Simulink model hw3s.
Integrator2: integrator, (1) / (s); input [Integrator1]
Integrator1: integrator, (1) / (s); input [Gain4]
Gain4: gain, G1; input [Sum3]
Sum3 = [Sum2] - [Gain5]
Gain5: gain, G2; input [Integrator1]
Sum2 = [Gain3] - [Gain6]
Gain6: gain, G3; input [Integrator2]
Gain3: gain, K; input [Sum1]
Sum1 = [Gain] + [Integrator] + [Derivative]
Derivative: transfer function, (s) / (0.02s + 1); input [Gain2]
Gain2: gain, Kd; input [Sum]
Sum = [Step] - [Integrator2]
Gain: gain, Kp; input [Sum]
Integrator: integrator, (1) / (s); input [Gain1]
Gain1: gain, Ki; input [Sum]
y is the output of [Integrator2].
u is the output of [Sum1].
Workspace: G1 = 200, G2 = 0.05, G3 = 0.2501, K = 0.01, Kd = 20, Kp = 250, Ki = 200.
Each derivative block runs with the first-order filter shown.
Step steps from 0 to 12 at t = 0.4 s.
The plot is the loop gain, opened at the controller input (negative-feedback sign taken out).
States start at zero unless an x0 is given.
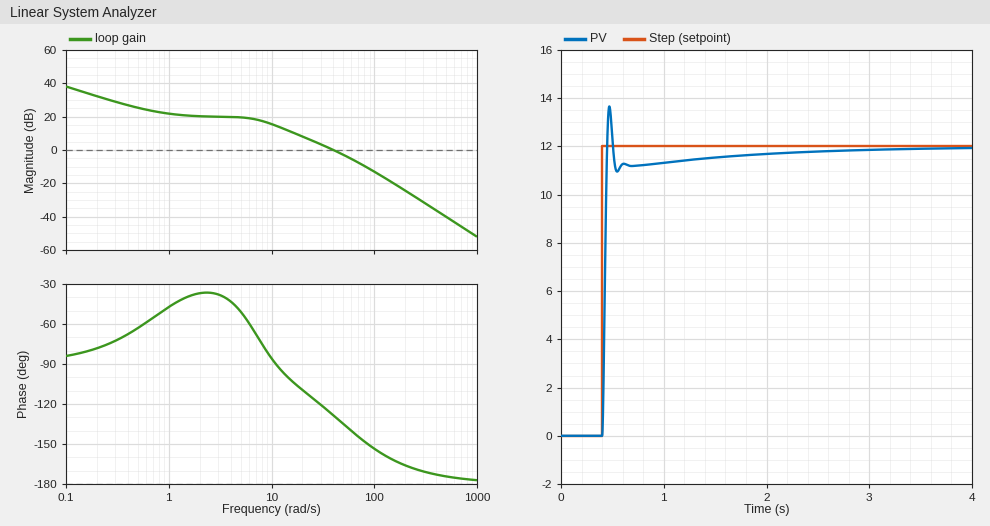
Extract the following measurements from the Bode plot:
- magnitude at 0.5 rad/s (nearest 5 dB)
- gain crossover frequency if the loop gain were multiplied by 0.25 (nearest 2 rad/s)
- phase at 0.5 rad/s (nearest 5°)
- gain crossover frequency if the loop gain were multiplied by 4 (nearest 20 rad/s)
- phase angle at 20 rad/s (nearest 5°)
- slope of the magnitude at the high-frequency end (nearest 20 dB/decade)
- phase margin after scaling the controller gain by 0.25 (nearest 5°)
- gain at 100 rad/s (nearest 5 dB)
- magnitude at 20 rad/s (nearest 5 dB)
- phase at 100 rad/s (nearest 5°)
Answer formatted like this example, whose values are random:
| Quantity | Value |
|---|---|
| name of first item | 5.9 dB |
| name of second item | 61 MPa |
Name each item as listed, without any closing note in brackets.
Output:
| Quantity | Value |
|---|---|
| magnitude at 0.5 rad/s | 25 dB |
| gain crossover frequency if the loop gain were multiplied by 0.25 | 14 rad/s |
| phase at 0.5 rad/s | -65° |
| gain crossover frequency if the loop gain were multiplied by 4 | 100 rad/s |
| phase angle at 20 rad/s | -110° |
| slope of the magnitude at the high-frequency end | -40 dB/decade |
| phase margin after scaling the controller gain by 0.25 | 80° |
| gain at 100 rad/s | -15 dB |
| magnitude at 20 rad/s | 10 dB |
| phase at 100 rad/s | -155° |
